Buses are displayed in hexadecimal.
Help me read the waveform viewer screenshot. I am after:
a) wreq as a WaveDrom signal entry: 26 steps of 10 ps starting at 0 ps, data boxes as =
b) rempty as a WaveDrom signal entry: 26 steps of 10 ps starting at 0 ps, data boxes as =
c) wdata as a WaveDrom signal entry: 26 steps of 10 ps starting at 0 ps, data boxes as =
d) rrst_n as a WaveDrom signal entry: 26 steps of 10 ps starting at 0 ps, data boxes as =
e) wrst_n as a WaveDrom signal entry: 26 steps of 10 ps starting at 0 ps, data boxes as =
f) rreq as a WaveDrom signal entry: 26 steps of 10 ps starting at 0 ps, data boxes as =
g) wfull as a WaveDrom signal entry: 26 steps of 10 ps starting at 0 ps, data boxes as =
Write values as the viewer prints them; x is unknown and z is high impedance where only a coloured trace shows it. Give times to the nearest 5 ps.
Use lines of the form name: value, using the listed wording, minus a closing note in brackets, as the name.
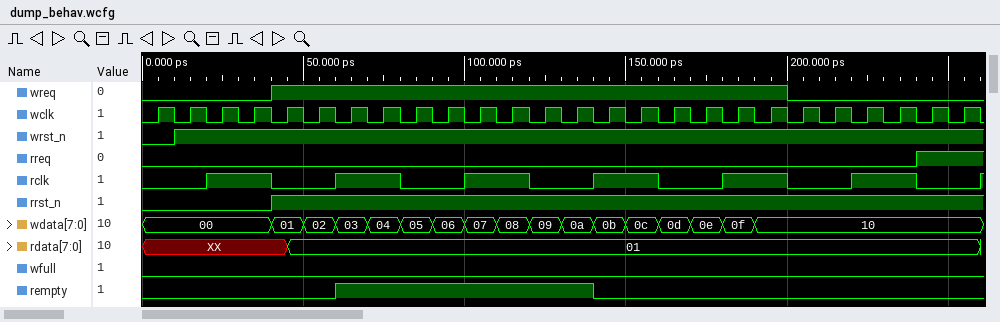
wreq as a WaveDrom signal entry: 26 steps of 10 ps starting at 0 ps, data boxes as =: {name: 'wreq', wave: '0...1...............0.....'}
rempty as a WaveDrom signal entry: 26 steps of 10 ps starting at 0 ps, data boxes as =: {name: 'rempty', wave: '0.....1.......0...........'}
wdata as a WaveDrom signal entry: 26 steps of 10 ps starting at 0 ps, data boxes as =: {name: 'wdata', wave: '=...================......', data: '00 01 02 03 04 05 06 07 08 09 0a 0b 0c 0d 0e 0f 10'}
rrst_n as a WaveDrom signal entry: 26 steps of 10 ps starting at 0 ps, data boxes as =: {name: 'rrst_n', wave: '0...1.....................'}
wrst_n as a WaveDrom signal entry: 26 steps of 10 ps starting at 0 ps, data boxes as =: {name: 'wrst_n', wave: '01........................'}
rreq as a WaveDrom signal entry: 26 steps of 10 ps starting at 0 ps, data boxes as =: {name: 'rreq', wave: '0.......................1.'}
wfull as a WaveDrom signal entry: 26 steps of 10 ps starting at 0 ps, data boxes as =: {name: 'wfull', wave: '0.........................'}
